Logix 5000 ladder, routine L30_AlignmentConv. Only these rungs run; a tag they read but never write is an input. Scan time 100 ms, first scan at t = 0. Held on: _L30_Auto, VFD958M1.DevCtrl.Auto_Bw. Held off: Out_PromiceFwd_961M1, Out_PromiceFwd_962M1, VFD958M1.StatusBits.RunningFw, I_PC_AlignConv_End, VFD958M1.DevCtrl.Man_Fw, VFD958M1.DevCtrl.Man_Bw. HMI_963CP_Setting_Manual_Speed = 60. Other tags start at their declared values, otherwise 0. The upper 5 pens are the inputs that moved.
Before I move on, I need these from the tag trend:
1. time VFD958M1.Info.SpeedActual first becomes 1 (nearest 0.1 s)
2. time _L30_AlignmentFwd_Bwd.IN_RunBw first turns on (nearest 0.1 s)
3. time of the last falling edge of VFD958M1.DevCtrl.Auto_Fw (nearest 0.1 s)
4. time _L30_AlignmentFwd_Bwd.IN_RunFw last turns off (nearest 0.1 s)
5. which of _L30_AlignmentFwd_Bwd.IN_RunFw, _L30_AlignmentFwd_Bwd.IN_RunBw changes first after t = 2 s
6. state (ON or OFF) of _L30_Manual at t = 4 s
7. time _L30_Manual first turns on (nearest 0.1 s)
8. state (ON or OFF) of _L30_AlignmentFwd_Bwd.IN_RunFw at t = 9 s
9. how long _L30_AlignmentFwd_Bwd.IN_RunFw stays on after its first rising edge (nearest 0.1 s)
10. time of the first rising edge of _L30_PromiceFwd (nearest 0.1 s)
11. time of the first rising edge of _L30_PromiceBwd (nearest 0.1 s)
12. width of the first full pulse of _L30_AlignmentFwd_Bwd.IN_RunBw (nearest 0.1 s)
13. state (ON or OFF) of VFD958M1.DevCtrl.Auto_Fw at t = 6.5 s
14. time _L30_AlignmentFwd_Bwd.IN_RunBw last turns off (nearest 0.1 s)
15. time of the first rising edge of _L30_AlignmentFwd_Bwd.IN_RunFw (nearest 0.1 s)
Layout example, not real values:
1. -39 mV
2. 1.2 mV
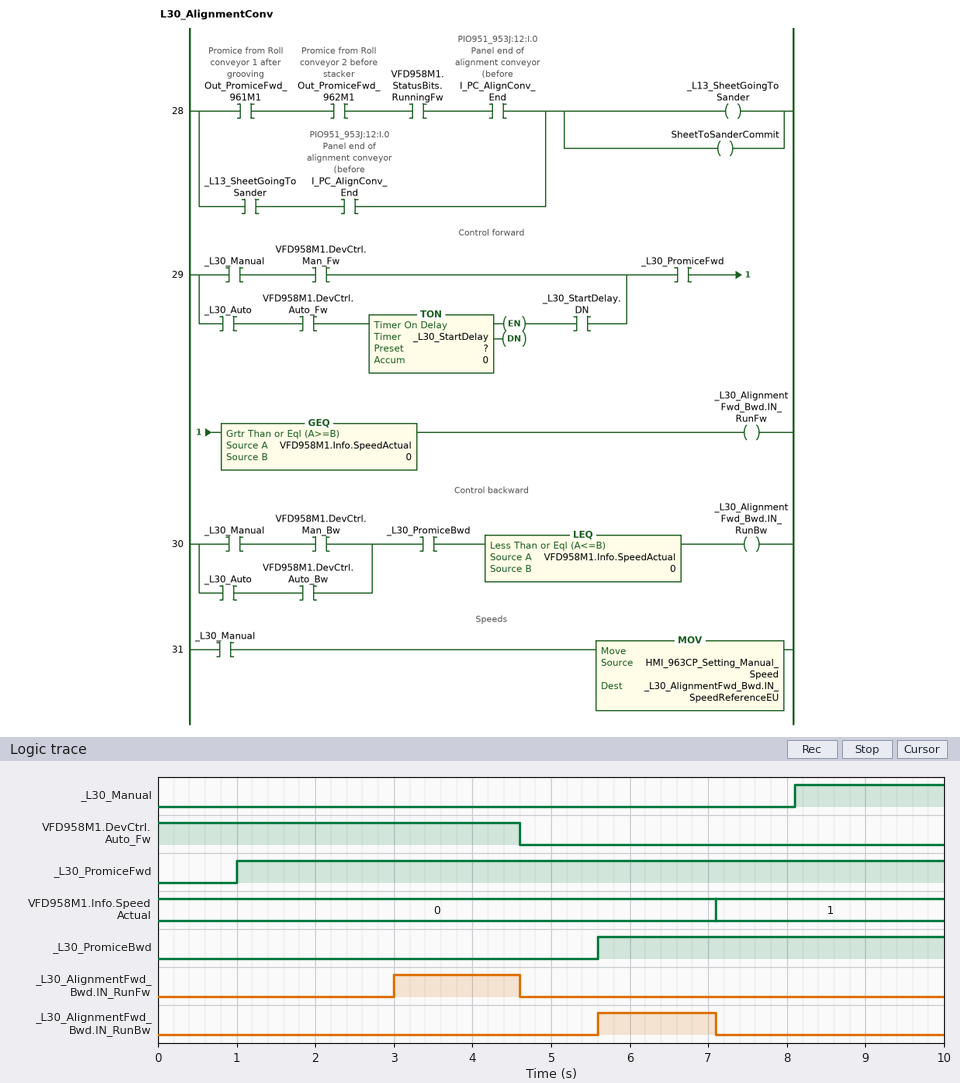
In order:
1. 7.1 s
2. 5.6 s
3. 4.6 s
4. 4.6 s
5. _L30_AlignmentFwd_Bwd.IN_RunFw
6. OFF
7. 8.1 s
8. OFF
9. 1.6 s
10. 1.0 s
11. 5.6 s
12. 1.5 s
13. OFF
14. 7.1 s
15. 3.0 s
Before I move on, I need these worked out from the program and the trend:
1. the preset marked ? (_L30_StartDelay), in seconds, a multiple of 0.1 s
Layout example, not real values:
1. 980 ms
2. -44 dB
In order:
1. 3.0 s
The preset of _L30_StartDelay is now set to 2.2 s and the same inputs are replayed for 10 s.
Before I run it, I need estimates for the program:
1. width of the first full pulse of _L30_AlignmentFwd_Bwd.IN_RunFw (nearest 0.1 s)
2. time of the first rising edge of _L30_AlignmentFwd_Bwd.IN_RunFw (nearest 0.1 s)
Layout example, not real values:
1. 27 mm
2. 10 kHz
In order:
1. 2.4 s
2. 2.2 s
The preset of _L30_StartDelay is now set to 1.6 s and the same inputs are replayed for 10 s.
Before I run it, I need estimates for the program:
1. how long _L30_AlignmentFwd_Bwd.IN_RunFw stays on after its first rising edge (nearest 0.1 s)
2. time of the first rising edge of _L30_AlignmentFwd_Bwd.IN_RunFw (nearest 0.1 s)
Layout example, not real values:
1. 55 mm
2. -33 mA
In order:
1. 3.0 s
2. 1.6 s
